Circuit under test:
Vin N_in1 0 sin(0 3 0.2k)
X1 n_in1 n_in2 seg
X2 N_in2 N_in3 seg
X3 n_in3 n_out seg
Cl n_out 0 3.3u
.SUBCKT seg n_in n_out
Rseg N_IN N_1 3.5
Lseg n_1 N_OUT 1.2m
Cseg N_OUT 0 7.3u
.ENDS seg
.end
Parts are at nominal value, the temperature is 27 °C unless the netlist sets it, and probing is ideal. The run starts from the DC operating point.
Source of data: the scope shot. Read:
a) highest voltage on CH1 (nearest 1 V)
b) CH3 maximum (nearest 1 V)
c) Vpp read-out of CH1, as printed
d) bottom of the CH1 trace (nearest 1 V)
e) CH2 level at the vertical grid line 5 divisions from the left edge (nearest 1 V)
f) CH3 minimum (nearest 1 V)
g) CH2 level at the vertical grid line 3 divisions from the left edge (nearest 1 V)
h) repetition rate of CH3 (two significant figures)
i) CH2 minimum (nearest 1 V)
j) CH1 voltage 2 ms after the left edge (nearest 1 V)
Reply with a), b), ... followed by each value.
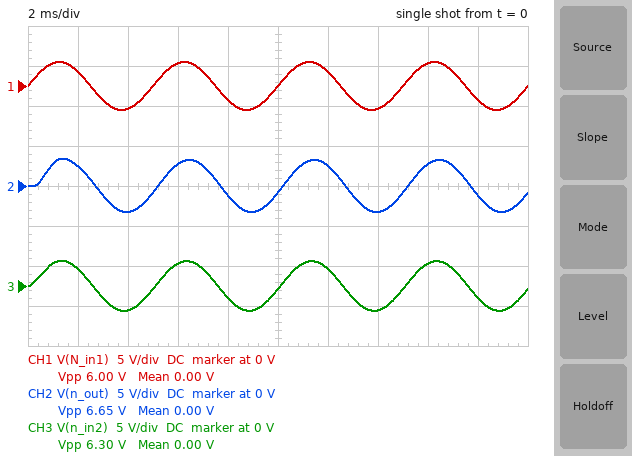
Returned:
a) 3 V
b) 3 V
c) 6.00 V
d) -3 V
e) -1 V
f) -3 V
g) 3 V
h) 200 Hz
i) -3 V
j) 2 V
